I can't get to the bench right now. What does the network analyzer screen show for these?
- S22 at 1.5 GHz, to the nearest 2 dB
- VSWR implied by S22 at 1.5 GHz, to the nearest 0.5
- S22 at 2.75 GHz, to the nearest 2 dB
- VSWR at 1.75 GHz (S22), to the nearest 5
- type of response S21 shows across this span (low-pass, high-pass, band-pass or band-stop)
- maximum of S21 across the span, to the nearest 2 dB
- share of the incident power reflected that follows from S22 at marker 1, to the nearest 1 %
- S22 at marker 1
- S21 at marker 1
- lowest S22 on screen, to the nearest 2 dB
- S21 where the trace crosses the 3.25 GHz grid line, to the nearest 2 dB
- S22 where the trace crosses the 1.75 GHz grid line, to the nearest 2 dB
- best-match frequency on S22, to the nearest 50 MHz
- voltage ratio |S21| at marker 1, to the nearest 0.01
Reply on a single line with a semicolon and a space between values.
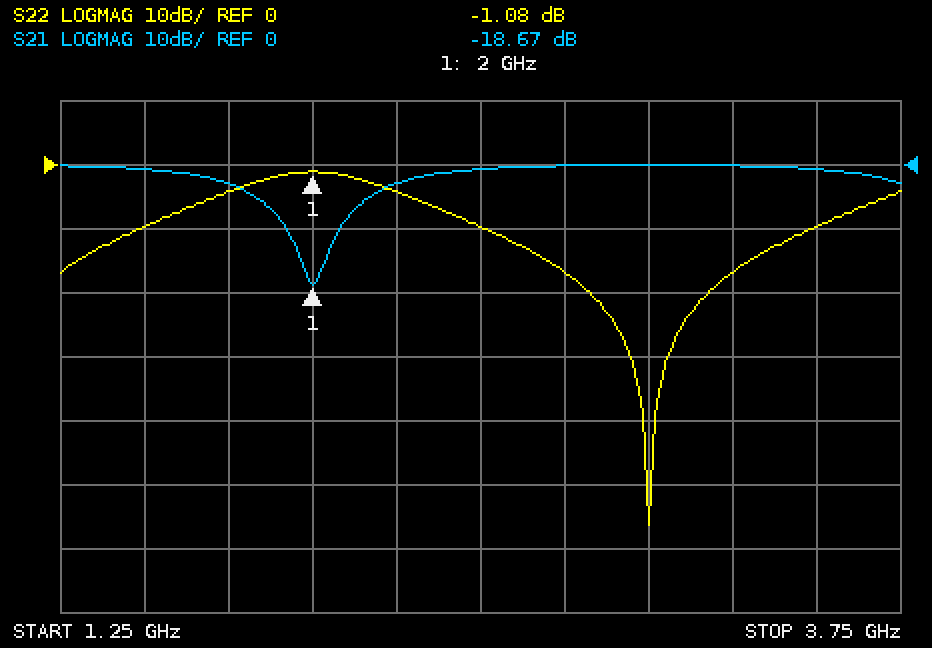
-10 dB; 2.0; -16 dB; 5; band-stop; 0 dB; 78 %; -1.08 dB; -18.67 dB; -56 dB; 0 dB; -4 dB; 3.00 GHz; 0.12
